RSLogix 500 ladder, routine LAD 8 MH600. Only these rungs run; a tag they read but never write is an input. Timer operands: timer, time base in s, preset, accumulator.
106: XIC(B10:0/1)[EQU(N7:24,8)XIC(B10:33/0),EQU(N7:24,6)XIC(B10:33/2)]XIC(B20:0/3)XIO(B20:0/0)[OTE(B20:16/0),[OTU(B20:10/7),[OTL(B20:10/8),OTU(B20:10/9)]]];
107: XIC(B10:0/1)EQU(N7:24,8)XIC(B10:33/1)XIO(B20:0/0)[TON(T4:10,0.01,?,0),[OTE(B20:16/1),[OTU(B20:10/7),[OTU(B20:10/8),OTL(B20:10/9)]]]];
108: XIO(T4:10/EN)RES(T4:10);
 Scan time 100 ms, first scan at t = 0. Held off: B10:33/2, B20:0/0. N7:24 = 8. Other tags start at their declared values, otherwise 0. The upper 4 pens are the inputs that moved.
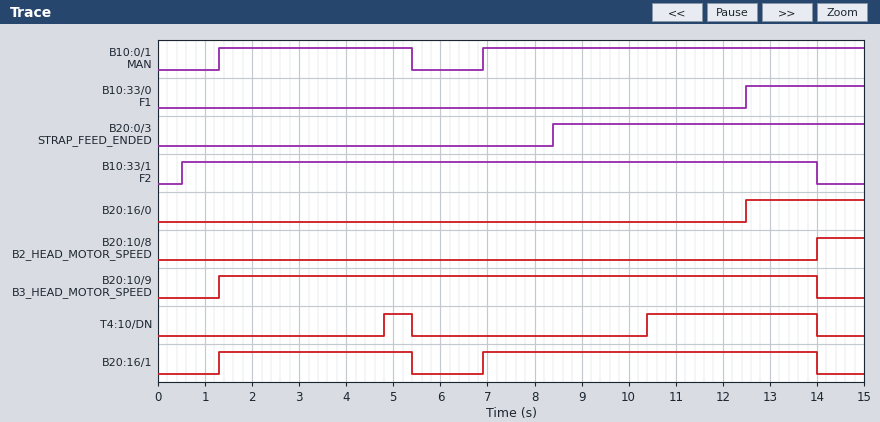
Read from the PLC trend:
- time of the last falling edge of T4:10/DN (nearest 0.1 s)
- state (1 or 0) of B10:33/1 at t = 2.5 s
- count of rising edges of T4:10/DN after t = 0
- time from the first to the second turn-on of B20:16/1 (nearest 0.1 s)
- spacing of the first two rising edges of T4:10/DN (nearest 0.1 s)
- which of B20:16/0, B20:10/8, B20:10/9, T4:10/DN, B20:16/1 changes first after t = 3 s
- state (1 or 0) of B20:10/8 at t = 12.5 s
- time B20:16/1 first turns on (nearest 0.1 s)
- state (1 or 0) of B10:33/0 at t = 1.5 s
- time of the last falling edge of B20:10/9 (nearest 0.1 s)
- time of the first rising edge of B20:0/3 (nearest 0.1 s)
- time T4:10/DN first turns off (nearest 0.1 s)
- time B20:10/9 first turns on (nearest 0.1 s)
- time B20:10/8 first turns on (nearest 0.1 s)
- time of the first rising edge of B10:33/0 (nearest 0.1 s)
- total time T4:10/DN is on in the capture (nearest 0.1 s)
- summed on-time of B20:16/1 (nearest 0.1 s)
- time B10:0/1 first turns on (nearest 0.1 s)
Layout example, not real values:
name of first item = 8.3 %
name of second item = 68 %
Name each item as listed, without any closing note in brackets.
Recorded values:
time of the last falling edge of T4:10/DN = 14.0 s
state (1 or 0) of B10:33/1 at t = 2.5 s = 1
count of rising edges of T4:10/DN after t = 0 = 2
time from the first to the second turn-on of B20:16/1 = 5.6 s
spacing of the first two rising edges of T4:10/DN = 5.6 s
which of B20:16/0, B20:10/8, B20:10/9, T4:10/DN, B20:16/1 changes first after t = 3 s = T4:10/DN
state (1 or 0) of B20:10/8 at t = 12.5 s = 0
time B20:16/1 first turns on = 1.3 s
state (1 or 0) of B10:33/0 at t = 1.5 s = 0
time of the last falling edge of B20:10/9 = 14.0 s
time of the first rising edge of B20:0/3 = 8.4 s
time T4:10/DN first turns off = 5.4 s
time B20:10/9 first turns on = 1.3 s
time B20:10/8 first turns on = 14.0 s
time of the first rising edge of B10:33/0 = 12.5 s
total time T4:10/DN is on in the capture = 4.2 s
summed on-time of B20:16/1 = 11.2 s
time B10:0/1 first turns on = 1.3 s
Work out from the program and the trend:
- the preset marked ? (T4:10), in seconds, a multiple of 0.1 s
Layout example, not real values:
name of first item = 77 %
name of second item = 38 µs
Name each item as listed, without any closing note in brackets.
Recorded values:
the preset marked ? (T4:10), in seconds, a multiple of 0.1 s = 3.5 s
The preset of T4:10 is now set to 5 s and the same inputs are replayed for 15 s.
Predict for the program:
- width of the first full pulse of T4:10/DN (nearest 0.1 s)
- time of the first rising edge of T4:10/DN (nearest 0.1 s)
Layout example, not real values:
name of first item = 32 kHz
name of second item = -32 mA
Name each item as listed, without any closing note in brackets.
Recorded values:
width of the first full pulse of T4:10/DN = 2.1 s
time of the first rising edge of T4:10/DN = 11.9 s
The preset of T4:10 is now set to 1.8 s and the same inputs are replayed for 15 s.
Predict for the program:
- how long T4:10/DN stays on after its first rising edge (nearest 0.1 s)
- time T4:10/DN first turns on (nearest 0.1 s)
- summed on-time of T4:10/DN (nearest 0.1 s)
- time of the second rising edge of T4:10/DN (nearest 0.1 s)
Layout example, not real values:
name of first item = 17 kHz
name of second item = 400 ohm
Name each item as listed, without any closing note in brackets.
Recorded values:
how long T4:10/DN stays on after its first rising edge = 2.3 s
time T4:10/DN first turns on = 3.1 s
summed on-time of T4:10/DN = 7.6 s
time of the second rising edge of T4:10/DN = 8.7 s
